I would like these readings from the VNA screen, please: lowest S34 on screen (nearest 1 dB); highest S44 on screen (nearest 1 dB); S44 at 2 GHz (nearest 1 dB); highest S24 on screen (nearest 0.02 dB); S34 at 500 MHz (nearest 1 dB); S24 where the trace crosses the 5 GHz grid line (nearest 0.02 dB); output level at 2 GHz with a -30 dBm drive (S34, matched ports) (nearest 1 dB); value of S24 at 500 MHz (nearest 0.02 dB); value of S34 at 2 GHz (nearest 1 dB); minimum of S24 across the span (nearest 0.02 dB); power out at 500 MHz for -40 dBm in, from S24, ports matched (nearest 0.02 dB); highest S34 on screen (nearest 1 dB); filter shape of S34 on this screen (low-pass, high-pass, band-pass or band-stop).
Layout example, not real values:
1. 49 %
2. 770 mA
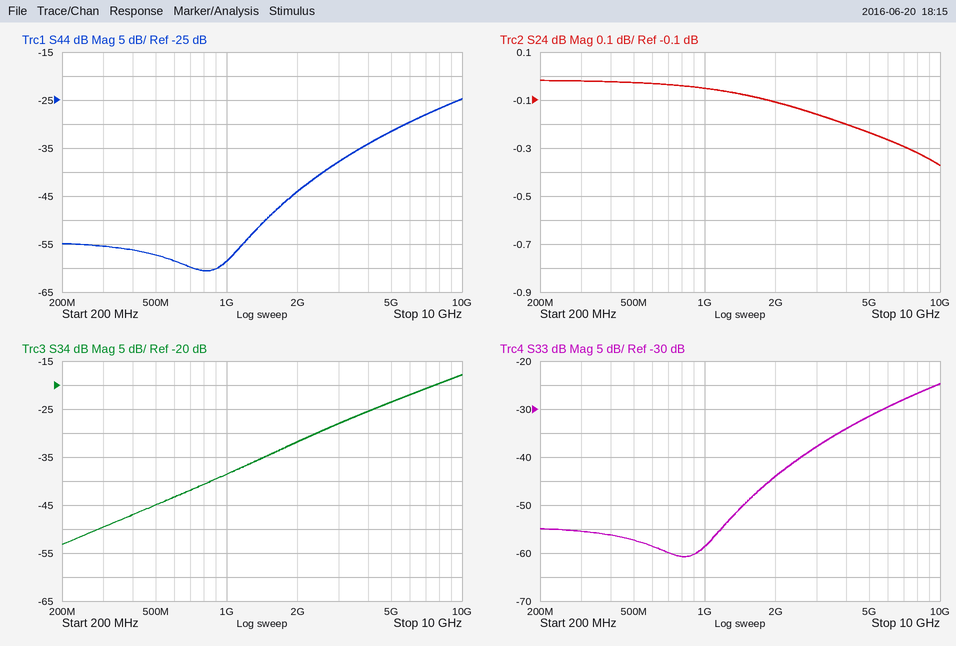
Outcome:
1. -53 dB
2. -25 dB
3. -44 dB
4. -0.02 dB
5. -45 dB
6. -0.24 dB
7. -62 dBm
8. -0.02 dB
9. -32 dB
10. -0.38 dB
11. -40.02 dBm
12. -18 dB
13. high-pass
